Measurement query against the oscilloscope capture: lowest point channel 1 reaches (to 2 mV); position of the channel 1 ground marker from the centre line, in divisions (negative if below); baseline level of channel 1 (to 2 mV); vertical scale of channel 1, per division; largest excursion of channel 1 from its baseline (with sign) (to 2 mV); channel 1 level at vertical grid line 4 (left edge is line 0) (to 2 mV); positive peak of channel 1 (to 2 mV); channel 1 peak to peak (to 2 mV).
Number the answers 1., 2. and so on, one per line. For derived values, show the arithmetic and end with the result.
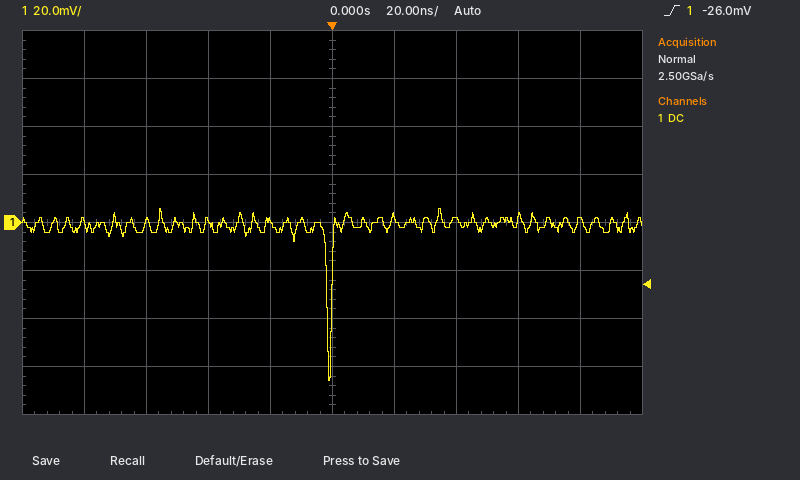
1. -66 mV
2. 0.0 div
3. 0 mV
4. 20 mV
5. -66 mV − (0 mV) = -66 mV
6. 0 mV
7. 6 mV
8. 6 mV − (-66 mV) = 72 mV
